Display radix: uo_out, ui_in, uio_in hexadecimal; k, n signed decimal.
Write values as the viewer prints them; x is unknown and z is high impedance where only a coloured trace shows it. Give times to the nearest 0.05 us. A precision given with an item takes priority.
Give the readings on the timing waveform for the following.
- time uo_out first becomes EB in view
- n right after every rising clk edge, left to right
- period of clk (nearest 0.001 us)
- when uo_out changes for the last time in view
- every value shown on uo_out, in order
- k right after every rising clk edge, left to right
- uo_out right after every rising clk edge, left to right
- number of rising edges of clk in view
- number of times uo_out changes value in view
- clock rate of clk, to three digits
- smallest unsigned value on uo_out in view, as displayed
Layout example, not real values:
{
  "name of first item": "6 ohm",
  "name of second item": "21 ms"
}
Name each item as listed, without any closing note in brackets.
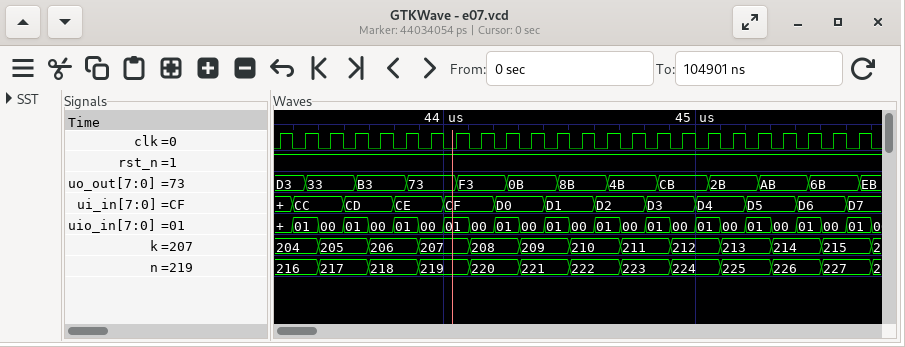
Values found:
{
  "time uo_out first becomes EB in view": "45.65 us",
  "n right after every rising clk edge, left to right": "216, 216, 217, 217, 218, 218, 219, 219, 220, 220, 221, 221, 222, 222, 223, 223, 224, 224, 225, 225, 226, 226, 227, 227",
  "period of clk": "0.1 us",
  "when uo_out changes for the last time in view": "45.65 us",
  "every value shown on uo_out, in order": "D3, 33, B3, 73, F3, 0B, 8B, 4B, CB, 2B, AB, 6B, EB",
  "k right after every rising clk edge, left to right": "204, 204, 205, 205, 206, 206, 207, 207, 208, 208, 209, 209, 210, 210, 211, 211, 212, 212, 213, 213, 214, 214, 215, 215",
  "uo_out right after every rising clk edge, left to right": "D3, 33, 33, B3, B3, 73, 73, F3, F3, 0B, 0B, 8B, 8B, 4B, 4B, CB, CB, 2B, 2B, AB, AB, 6B, 6B, EB",
  "number of rising edges of clk in view": "24",
  "number of times uo_out changes value in view": "12",
  "clock rate of clk, to three digits": "10.0 MHz",
  "smallest unsigned value on uo_out in view, as displayed": "0B"
}
